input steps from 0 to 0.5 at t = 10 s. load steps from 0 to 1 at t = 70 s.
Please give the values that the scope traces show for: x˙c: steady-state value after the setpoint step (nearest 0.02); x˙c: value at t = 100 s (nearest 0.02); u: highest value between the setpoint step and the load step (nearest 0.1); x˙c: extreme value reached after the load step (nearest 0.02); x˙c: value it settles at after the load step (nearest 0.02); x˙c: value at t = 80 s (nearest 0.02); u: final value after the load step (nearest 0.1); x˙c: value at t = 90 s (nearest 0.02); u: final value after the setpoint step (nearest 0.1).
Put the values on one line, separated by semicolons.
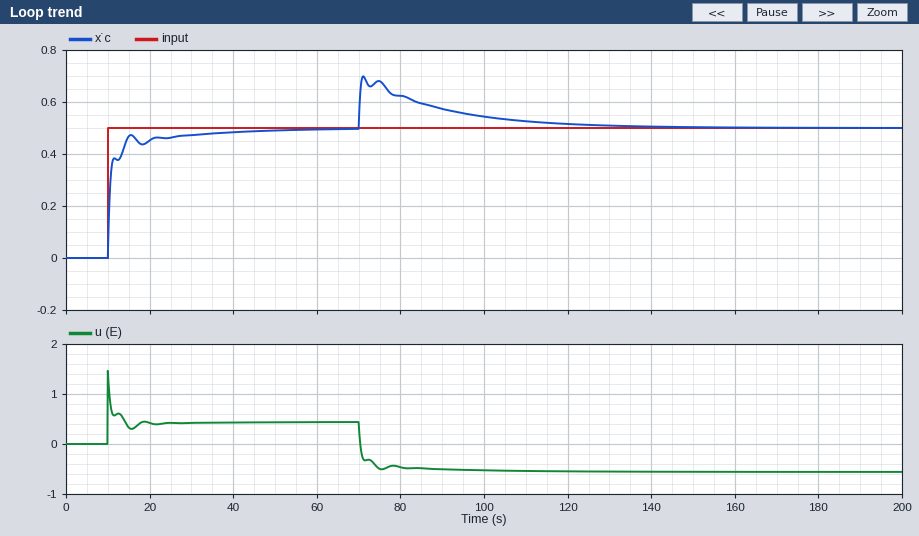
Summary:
0.50; 0.54; 1.5; 0.70; 0.50; 0.62; -0.6; 0.58; 0.4
